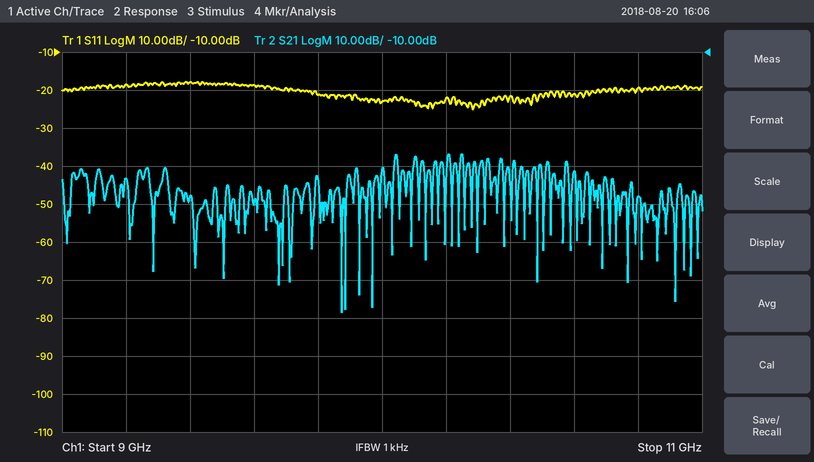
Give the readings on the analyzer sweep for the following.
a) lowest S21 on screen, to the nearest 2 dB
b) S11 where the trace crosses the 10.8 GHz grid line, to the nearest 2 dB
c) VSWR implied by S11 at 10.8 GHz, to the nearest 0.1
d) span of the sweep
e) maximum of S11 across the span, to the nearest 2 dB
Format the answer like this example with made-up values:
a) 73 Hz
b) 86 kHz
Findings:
a) -78 dB
b) -20 dB
c) 1.2
d) 2 GHz
e) -18 dB
